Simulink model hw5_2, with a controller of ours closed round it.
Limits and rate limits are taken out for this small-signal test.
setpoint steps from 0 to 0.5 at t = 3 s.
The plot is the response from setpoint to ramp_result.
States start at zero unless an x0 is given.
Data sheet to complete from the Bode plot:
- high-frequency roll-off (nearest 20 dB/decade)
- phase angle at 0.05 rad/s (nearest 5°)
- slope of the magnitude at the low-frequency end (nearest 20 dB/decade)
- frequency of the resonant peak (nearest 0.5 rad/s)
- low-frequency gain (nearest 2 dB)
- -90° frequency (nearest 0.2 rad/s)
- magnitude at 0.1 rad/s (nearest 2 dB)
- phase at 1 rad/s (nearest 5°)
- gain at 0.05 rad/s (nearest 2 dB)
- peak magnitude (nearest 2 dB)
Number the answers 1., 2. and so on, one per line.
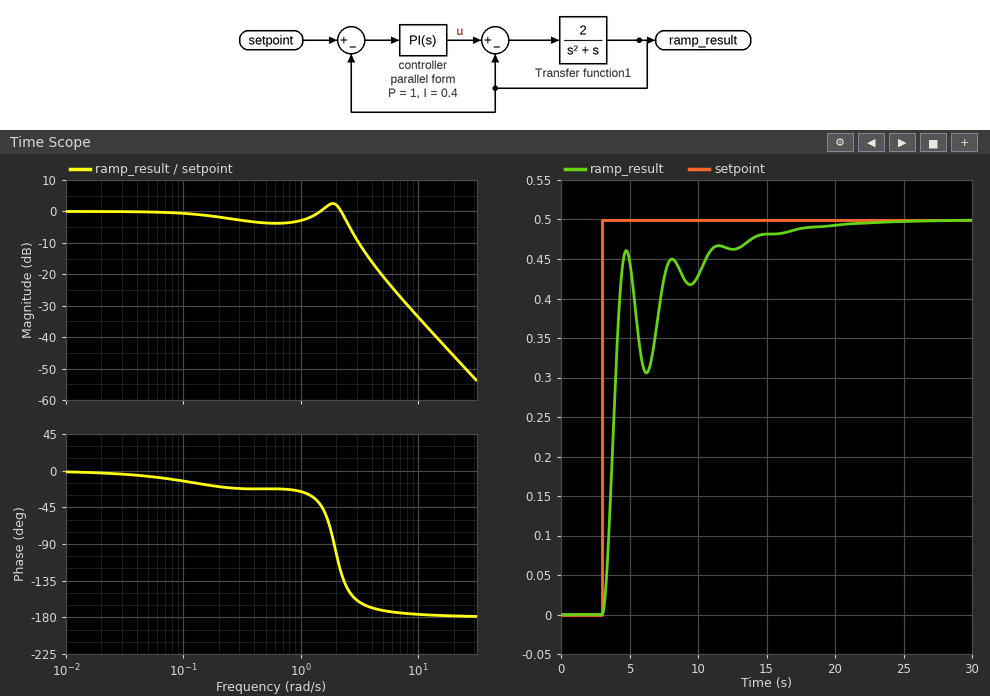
1. -40 dB/decade
2. -5°
3. 0 dB/decade
4. 2.0 rad/s
5. 0 dB
6. 2.0 rad/s
7. 0 dB
8. -25°
9. 0 dB
10. 2 dB
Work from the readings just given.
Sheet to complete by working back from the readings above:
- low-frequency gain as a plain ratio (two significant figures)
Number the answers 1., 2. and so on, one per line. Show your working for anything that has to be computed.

1. 10^(0 / 20) = 1.0
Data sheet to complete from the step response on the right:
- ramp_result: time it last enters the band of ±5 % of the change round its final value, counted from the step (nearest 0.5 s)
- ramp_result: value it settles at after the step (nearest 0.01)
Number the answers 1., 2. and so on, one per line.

1. 11.0 s
2. 0.50
